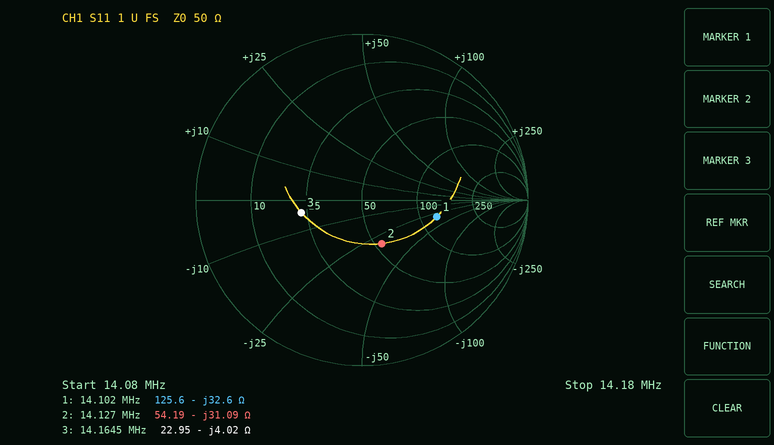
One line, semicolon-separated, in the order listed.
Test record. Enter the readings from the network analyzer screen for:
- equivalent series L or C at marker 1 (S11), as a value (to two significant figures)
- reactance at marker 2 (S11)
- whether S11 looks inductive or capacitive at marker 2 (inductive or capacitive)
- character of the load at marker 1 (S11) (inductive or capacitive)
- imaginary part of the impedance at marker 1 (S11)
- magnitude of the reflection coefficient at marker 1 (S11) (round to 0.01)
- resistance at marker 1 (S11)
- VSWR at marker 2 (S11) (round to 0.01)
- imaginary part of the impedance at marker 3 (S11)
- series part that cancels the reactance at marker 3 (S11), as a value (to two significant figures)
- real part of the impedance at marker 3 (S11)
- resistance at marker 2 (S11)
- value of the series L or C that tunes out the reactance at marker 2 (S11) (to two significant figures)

350 pF; -31.09 Ω; capacitive; capacitive; -32.6 Ω; 0.46; 125.6 Ω; 1.81; -4.02 Ω; 45 nH; 22.95 Ω; 54.19 Ω; 350 nH
